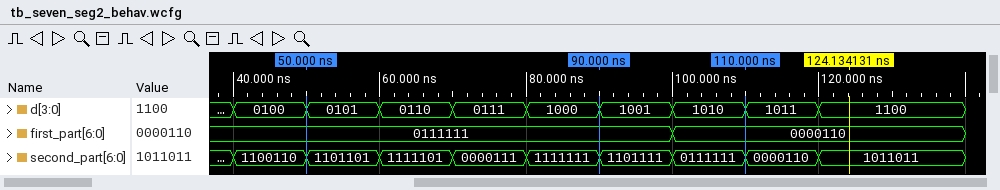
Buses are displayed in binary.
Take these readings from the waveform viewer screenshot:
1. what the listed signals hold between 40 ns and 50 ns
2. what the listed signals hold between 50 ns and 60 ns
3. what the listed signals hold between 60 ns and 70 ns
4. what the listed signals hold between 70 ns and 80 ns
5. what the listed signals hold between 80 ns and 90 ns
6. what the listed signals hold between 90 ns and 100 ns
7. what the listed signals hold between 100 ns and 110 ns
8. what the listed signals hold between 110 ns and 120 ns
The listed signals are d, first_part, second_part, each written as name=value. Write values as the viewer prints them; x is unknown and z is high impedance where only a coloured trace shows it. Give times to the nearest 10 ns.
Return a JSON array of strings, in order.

["d=0100, first_part=0111111, second_part=1100110", "d=0101, first_part=0111111, second_part=1101101", "d=0110, first_part=0111111, second_part=1111101", "d=0111, first_part=0111111, second_part=0000111", "d=1000, first_part=0111111, second_part=1111111", "d=1001, first_part=0111111, second_part=1101111", "d=1010, first_part=0000110, second_part=0111111", "d=1011, first_part=0000110, second_part=0000110"]
